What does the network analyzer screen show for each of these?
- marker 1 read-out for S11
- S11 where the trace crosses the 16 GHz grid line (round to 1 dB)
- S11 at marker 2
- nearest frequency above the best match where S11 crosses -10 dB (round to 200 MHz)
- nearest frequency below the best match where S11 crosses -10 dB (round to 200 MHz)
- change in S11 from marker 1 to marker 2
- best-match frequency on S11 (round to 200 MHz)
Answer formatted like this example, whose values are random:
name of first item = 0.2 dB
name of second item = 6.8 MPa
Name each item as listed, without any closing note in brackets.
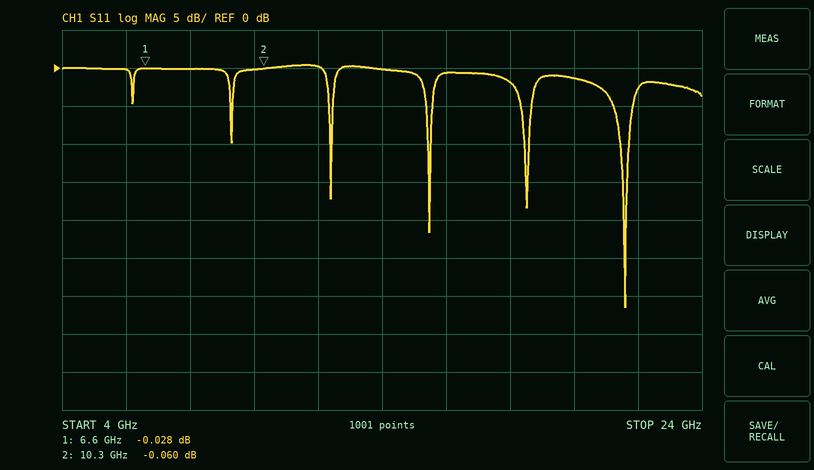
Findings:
marker 1 read-out for S11 = -0.028 dB
S11 where the trace crosses the 16 GHz grid line = -1 dB
S11 at marker 2 = -0.060 dB
nearest frequency above the best match where S11 crosses -10 dB = 21.8 GHz
nearest frequency below the best match where S11 crosses -10 dB = 21.4 GHz
change in S11 from marker 1 to marker 2 = -0.032 dB
best-match frequency on S11 = 21.6 GHz
